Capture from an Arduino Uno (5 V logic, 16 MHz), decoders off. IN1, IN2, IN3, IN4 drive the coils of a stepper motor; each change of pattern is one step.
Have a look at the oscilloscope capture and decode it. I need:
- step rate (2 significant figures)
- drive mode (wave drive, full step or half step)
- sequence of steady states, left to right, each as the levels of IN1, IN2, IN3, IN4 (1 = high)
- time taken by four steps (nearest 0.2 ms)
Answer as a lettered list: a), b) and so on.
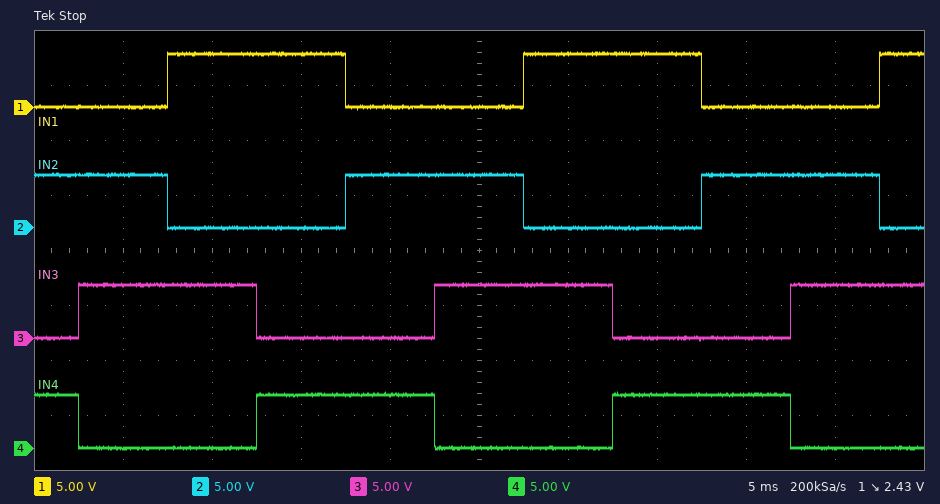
a) 200 steps/s
b) full step
c) 0101 0110 1010 1001 0101 0110 1010 1001 0101 0110 1010
d) 20.0 ms
